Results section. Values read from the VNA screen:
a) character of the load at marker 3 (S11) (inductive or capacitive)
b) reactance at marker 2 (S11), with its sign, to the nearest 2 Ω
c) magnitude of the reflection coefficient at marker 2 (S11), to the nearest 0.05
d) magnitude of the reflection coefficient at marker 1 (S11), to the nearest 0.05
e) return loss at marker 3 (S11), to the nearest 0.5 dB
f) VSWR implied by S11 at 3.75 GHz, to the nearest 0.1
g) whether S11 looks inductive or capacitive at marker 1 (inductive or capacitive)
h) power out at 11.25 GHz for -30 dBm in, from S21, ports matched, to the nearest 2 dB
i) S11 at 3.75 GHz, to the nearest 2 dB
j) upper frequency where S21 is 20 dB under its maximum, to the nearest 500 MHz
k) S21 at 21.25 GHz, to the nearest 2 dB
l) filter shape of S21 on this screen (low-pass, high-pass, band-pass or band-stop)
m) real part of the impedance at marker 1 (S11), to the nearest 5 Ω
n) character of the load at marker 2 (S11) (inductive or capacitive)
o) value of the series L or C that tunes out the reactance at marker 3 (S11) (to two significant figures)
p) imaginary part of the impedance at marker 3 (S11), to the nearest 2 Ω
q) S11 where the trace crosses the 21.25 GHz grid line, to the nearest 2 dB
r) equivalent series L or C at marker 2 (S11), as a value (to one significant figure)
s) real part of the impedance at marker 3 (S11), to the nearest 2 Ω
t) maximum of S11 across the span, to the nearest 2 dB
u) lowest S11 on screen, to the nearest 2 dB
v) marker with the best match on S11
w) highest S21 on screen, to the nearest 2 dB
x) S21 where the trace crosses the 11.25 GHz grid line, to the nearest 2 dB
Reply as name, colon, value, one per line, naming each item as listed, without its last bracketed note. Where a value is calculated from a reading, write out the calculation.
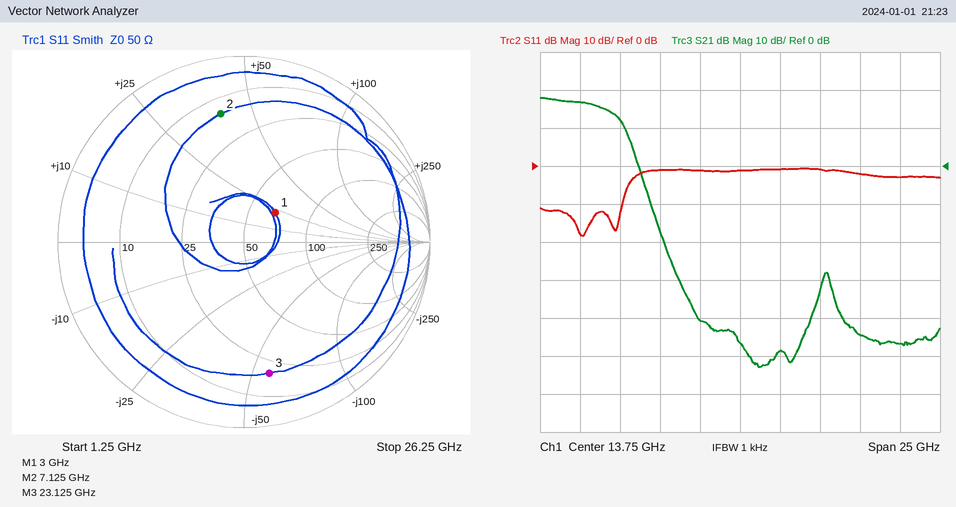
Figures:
character of the load at marker 3 (S11): capacitive
reactance at marker 2 (S11), with its sign, to the nearest 2 Ω: +40 Ω
magnitude of the reflection coefficient at marker 2 (S11), to the nearest 0.05: 0.70
magnitude of the reflection coefficient at marker 1 (S11), to the nearest 0.05: 0.25
return loss at marker 3 (S11), to the nearest 0.5 dB: 3.0 dB
VSWR implied by S11 at 3.75 GHz, to the nearest 0.1: |Γ| = 10^(-18/20) = 0.1259; VSWR = (1 + 0.1259)/(1 − 0.1259) ≈ 1.3
whether S11 looks inductive or capacitive at marker 1: inductive
power out at 11.25 GHz for -30 dBm in, from S21, ports matched, to the nearest 2 dB: -30 dBm + (-40 dB) = -70 dBm
S11 at 3.75 GHz, to the nearest 2 dB: -18 dB
upper frequency where S21 is 20 dB under its maximum, to the nearest 500 MHz: 7.5 GHz
S21 at 21.25 GHz, to the nearest 2 dB: -44 dB
filter shape of S21 on this screen: low-pass
real part of the impedance at marker 1 (S11), to the nearest 5 Ω: 65 Ω
character of the load at marker 2 (S11): inductive
value of the series L or C that tunes out the reactance at marker 3 (S11): L = 56 Ω/(2π × 23.125 GHz) ≈ 385 pH, so 390 pH to two significant figures
imaginary part of the impedance at marker 3 (S11), to the nearest 2 Ω: -56 Ω
S11 where the trace crosses the 21.25 GHz grid line, to the nearest 2 dB: -2 dB
equivalent series L or C at marker 2 (S11), as a value: L = 40 Ω/(2π × 7.125 GHz) ≈ 894 pH, so 900 pH to one significant figure
real part of the impedance at marker 3 (S11), to the nearest 2 Ω: 20 Ω
maximum of S11 across the span, to the nearest 2 dB: 0 dB
lowest S11 on screen, to the nearest 2 dB: -18 dB
marker with the best match on S11: marker 1
highest S21 on screen, to the nearest 2 dB: 18 dB
S21 where the trace crosses the 11.25 GHz grid line, to the nearest 2 dB: -40 dB
